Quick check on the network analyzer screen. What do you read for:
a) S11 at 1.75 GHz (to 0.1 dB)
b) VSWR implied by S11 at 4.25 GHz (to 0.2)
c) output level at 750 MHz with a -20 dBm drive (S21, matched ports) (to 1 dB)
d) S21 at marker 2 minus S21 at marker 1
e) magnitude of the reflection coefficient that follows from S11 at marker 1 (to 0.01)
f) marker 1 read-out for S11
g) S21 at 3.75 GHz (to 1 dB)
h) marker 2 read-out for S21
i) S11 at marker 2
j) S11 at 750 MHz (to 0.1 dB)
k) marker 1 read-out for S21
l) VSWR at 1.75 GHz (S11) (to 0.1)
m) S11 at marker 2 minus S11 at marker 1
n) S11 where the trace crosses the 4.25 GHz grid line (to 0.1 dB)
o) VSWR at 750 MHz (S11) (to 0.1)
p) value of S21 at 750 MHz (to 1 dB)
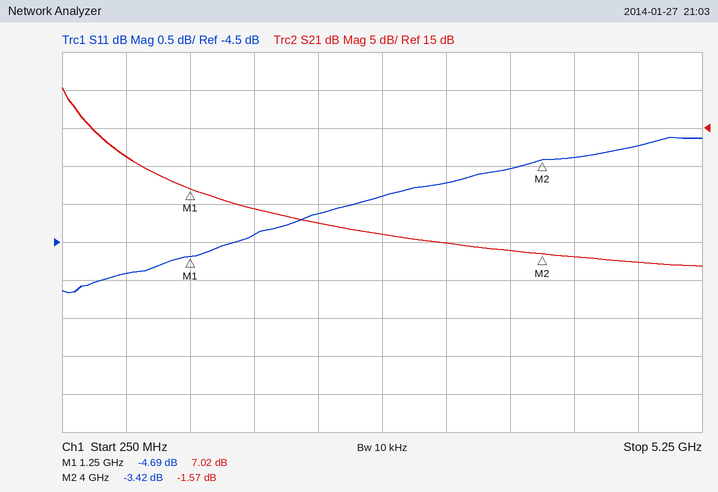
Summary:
-4.4 dB
5.2
-9 dBm
-8.59 dB
0.58
-4.69 dB
-1 dB
-1.57 dB
-3.42 dB
-4.9 dB
7.02 dB
4.0
1.27 dB
-3.4 dB
3.6
11 dB
